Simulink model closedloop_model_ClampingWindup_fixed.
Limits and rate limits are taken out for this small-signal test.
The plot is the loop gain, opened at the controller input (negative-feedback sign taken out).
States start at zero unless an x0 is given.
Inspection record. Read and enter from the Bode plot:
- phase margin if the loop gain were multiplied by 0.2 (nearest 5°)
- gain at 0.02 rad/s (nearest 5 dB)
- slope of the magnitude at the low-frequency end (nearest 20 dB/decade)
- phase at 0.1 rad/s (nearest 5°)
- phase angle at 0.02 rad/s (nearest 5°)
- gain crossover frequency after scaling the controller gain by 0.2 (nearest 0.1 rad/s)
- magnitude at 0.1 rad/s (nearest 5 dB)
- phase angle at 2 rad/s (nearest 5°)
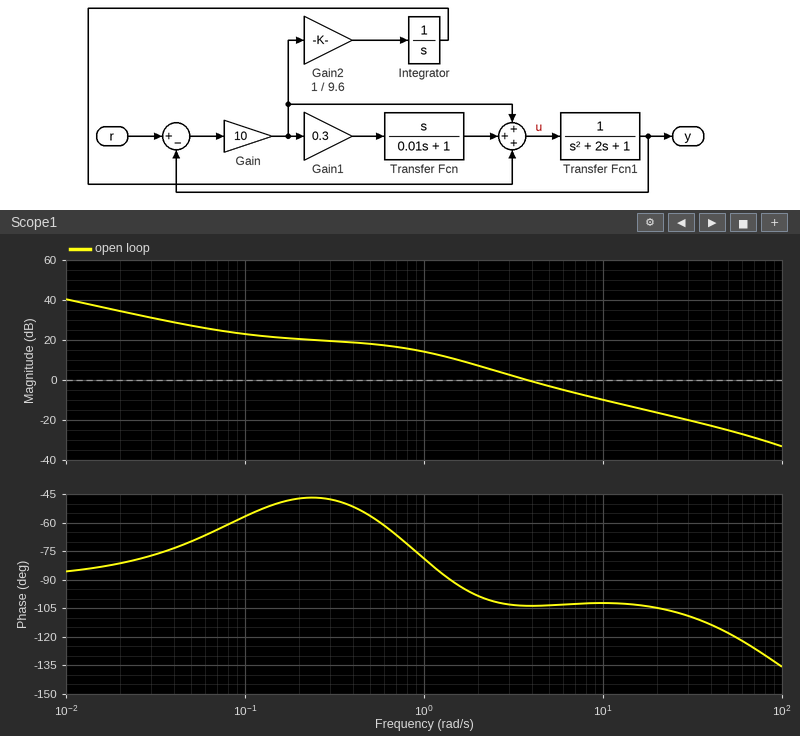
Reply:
100°
35 dB
-20 dB/decade
-55°
-80°
1.0 rad/s
25 dB
-100°
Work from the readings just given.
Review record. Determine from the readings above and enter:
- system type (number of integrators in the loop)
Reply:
1
